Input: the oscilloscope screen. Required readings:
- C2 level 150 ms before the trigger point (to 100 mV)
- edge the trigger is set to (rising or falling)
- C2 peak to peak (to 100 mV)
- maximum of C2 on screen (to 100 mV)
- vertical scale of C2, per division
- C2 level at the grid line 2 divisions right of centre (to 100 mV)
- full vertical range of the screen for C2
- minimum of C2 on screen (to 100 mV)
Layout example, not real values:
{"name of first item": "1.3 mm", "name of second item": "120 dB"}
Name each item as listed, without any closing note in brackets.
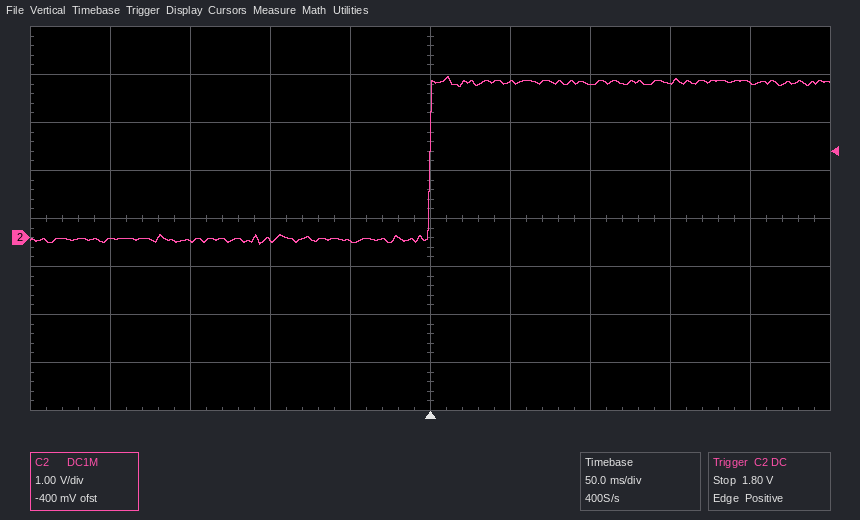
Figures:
{"C2 level 150 ms before the trigger point": "-100 mV", "edge the trigger is set to": "rising", "C2 peak to peak": "3.5 V", "maximum of C2 on screen": "3.4 V", "vertical scale of C2, per division": "1 V", "C2 level at the grid line 2 divisions right of centre": "3.2 V", "full vertical range of the screen for C2": "8 V", "minimum of C2 on screen": "-100 mV"}
